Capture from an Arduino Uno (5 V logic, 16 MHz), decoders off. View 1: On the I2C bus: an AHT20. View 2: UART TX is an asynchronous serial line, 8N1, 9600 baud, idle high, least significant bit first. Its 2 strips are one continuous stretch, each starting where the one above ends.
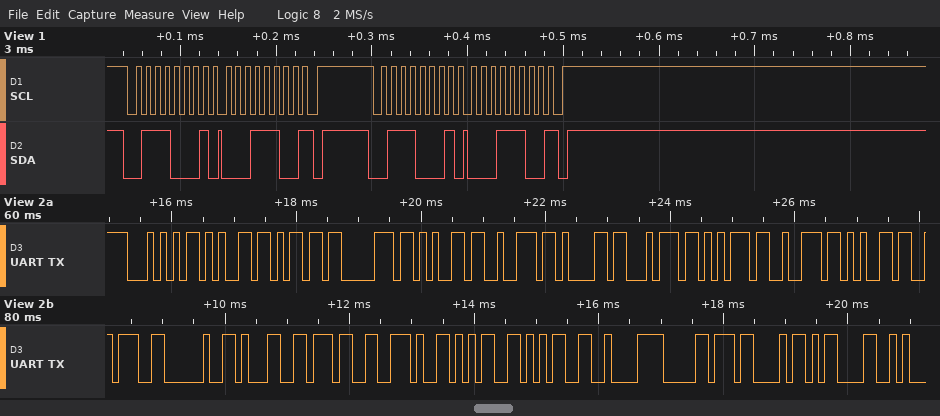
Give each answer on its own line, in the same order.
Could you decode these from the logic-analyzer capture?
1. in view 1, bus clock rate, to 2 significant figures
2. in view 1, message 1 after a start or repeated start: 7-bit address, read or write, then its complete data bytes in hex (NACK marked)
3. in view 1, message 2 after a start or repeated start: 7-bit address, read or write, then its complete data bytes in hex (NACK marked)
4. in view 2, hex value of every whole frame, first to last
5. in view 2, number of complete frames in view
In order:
100 kHz
0x38 read: 1C NACK
0x38 read: 1C NACK
54 65 6D 70 65 72 61 74 75 72 65 3A 20 31 37 2E 35 35 C2 B0 43 0D
22
